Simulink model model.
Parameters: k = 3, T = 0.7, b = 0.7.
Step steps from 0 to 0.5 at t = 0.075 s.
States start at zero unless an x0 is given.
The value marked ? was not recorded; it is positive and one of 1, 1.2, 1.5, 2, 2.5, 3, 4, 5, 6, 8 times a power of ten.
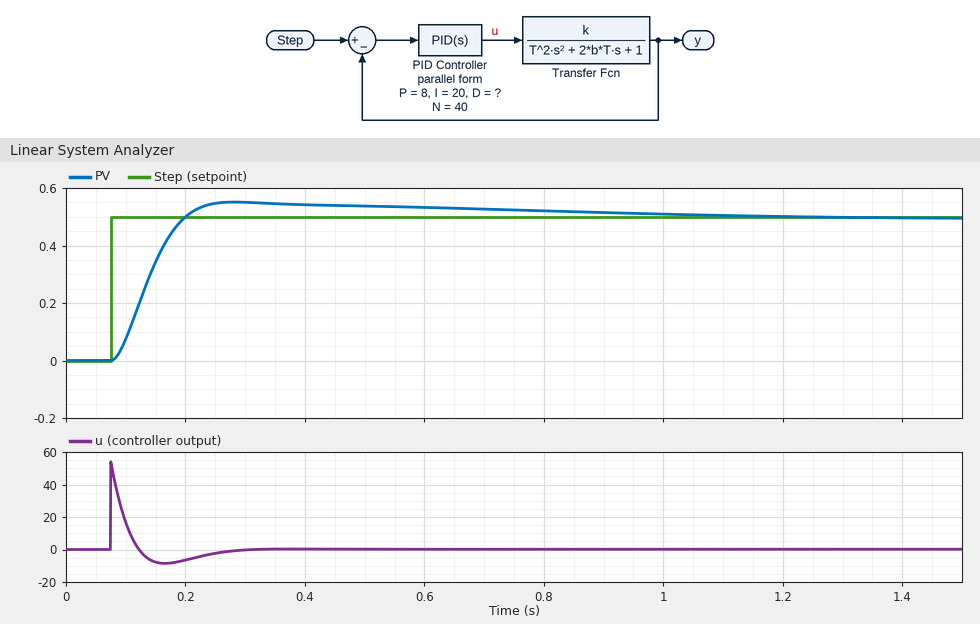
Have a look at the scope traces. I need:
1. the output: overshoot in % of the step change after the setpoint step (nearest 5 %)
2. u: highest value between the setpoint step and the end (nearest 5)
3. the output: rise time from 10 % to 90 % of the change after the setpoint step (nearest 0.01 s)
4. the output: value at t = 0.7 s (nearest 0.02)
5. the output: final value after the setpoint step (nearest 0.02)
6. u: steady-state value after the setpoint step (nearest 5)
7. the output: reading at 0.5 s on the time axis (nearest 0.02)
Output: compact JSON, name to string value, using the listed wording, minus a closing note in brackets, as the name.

{"the output: overshoot in % of the step change after the setpoint step": "10 %", "u: highest value between the setpoint step and the end": "55", "the output: rise time from 10 % to 90 % of the change after the setpoint step": "0.08 s", "the output: value at t = 0.7 s": "0.52", "the output: final value after the setpoint step": "0.50", "u: steady-state value after the setpoint step": "0", "the output: reading at 0.5 s on the time axis": "0.54"}
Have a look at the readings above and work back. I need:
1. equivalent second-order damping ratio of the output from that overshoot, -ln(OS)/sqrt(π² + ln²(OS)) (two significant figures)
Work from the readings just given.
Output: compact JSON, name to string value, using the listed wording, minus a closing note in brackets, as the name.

{"equivalent second-order damping ratio of the output from that overshoot, -ln(OS)/sqrt(π² + ln²(OS))": "0.59"}
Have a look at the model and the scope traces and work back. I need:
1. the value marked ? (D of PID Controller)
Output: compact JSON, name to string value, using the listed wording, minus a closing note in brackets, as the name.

{"the value marked ?": "2.5"}
